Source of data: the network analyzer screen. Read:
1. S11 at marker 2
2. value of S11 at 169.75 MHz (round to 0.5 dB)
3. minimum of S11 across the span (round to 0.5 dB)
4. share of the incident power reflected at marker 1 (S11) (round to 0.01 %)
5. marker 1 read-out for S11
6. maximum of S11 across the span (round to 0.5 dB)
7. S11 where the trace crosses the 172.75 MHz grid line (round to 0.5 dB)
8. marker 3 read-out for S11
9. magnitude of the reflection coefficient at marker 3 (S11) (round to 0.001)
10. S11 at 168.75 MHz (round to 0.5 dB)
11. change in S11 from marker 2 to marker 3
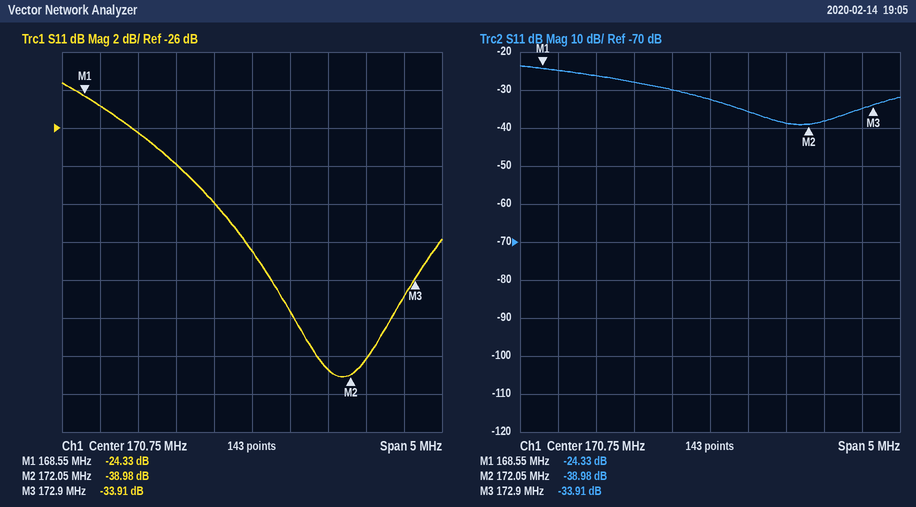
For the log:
-38.98 dB
-28.0 dB
-39.0 dB
0.37 %
-24.33 dB
-23.5 dB
-35.0 dB
-33.91 dB
0.020
-25.0 dB
5.07 dB
